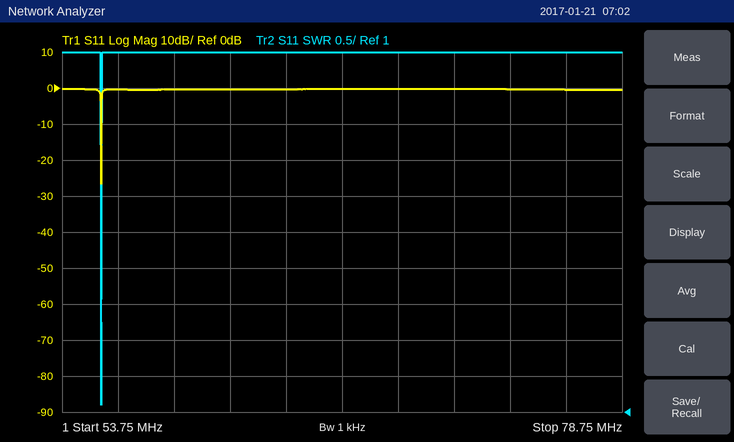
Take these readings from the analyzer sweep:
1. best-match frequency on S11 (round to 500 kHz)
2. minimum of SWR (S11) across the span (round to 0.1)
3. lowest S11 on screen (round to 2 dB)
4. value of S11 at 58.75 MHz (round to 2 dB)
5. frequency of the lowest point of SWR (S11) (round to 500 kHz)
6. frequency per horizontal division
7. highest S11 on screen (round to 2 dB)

55.5 MHz
1.1
-26 dB
0 dB
55.5 MHz
2.5 MHz
0 dB
